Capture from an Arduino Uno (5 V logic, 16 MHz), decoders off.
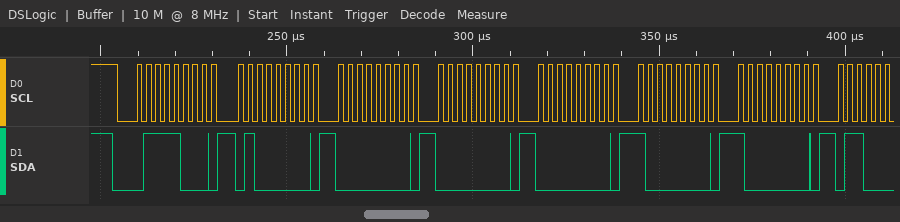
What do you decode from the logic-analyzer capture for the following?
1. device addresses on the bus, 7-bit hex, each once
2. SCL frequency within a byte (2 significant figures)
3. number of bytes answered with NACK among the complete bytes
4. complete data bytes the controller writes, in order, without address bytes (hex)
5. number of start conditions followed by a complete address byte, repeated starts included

0x3C
400 kHz
0
40 00 00 00 80 80
1
